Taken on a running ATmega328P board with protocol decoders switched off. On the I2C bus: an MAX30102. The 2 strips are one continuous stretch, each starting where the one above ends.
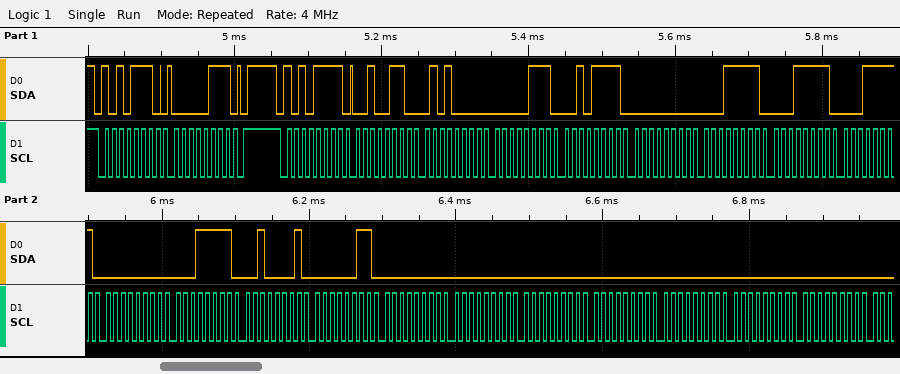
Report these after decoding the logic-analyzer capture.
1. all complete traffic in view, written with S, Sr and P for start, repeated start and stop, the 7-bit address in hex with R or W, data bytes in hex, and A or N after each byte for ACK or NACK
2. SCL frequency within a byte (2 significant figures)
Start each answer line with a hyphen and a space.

- S 57W A 07 A P S 57R A 26 A 50 A 07 A 2F A 00 A 1F A 1F A 1F A 00 A 1F A 21 A 03 A 00 A 00 A 00 A 00 A 00 A 00 A 00 A
- 100 kHz
